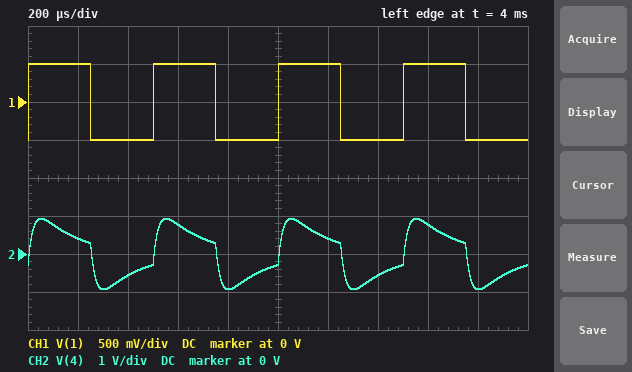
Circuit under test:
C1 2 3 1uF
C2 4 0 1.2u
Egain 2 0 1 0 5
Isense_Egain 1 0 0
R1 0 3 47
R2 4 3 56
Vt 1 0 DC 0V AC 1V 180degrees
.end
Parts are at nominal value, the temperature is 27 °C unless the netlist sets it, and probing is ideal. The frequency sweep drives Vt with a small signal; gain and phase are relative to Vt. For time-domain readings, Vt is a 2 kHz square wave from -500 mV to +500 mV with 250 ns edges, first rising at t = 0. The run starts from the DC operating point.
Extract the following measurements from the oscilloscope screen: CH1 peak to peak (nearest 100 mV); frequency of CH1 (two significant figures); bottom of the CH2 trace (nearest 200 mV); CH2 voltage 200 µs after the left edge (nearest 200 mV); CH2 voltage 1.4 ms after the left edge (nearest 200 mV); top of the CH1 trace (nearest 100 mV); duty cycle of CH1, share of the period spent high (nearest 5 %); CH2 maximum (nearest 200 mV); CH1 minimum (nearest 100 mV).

1.0 V
2.0 kHz
-1.0 V
400 mV
-600 mV
500 mV
50 %
1.0 V
-500 mV
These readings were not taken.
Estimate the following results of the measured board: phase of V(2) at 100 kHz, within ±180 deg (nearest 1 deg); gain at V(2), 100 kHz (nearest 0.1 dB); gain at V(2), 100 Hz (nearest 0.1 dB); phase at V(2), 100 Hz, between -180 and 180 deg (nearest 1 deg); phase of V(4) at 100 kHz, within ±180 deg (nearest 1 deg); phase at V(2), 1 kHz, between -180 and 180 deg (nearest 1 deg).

0 deg
14.0 dB
14.0 dB
0 deg
-85 deg
0 deg
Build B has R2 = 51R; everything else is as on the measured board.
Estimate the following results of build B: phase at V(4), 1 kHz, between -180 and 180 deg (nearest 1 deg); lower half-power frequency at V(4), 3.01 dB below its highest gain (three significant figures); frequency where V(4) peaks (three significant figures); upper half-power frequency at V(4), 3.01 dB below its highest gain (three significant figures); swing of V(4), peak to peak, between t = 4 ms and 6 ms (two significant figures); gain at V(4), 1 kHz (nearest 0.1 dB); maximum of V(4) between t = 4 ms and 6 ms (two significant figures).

41 deg
882 Hz
2.97 kHz
9.99 kHz
2.0 V
0.7 dB
980 mV
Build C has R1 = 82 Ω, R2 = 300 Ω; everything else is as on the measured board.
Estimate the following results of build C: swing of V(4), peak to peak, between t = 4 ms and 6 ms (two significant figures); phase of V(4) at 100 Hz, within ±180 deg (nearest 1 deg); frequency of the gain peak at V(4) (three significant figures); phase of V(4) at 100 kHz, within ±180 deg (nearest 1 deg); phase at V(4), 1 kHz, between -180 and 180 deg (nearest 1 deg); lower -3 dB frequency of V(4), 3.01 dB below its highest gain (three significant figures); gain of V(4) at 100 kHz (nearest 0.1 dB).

740 mV
71 deg
926 Hz
-88 deg
-3 deg
270 Hz
-33.1 dB
